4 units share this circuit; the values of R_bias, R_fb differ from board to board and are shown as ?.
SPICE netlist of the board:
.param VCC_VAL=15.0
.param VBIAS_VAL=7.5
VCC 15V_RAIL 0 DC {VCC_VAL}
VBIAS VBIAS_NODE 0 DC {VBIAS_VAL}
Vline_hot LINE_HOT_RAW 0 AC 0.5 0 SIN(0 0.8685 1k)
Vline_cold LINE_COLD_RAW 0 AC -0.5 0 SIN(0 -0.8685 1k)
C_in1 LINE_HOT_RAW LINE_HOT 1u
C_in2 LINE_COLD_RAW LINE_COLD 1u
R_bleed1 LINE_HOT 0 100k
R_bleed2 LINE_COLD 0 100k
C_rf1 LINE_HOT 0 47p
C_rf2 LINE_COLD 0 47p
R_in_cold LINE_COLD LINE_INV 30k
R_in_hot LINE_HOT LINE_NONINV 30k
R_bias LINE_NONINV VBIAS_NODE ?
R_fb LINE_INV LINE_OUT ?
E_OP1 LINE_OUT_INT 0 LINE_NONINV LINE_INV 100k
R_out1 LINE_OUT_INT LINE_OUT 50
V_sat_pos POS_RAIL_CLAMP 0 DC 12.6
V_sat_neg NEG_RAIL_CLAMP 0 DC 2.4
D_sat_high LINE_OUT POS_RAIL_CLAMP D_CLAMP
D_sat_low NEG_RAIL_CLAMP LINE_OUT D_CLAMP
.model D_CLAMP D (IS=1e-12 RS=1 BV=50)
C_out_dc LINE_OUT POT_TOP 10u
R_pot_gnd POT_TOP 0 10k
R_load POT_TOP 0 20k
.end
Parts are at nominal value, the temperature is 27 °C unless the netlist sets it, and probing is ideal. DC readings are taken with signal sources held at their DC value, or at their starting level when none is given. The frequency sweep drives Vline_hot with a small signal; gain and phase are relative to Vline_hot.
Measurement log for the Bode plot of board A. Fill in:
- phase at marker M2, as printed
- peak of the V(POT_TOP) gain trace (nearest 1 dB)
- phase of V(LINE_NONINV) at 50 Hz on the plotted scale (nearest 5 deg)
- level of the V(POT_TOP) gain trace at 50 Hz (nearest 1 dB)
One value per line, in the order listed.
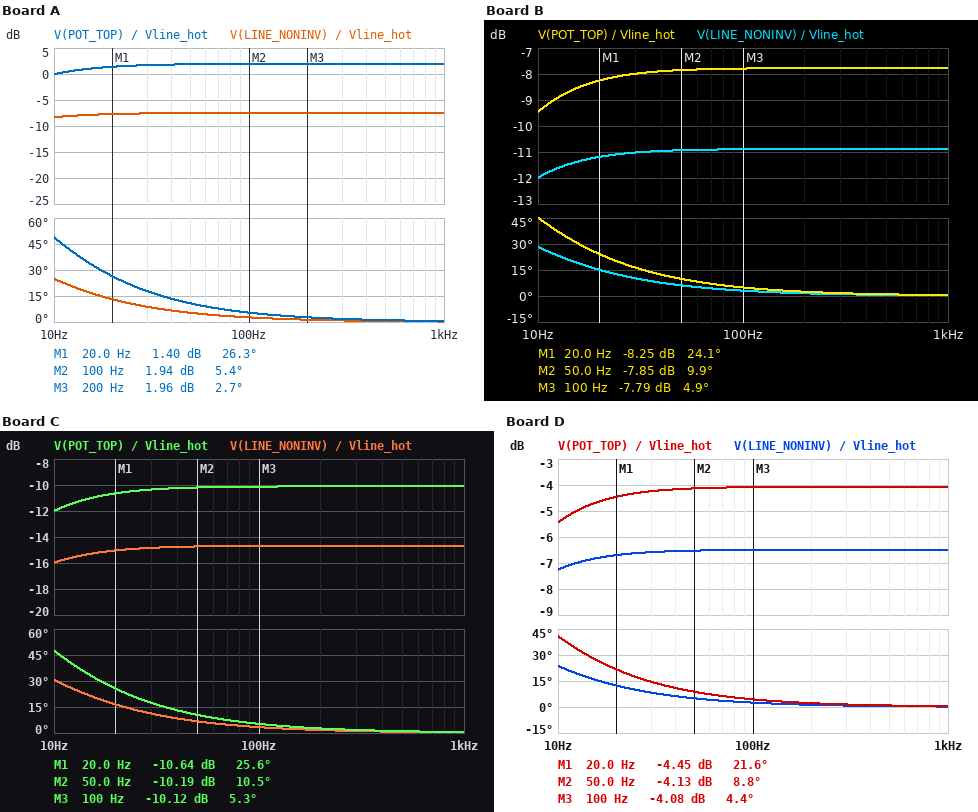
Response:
5.4 deg
2 dB
5 deg
2 dB
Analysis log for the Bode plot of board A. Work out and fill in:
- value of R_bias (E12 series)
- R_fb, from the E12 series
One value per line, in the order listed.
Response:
22 kΩ
27 kΩ
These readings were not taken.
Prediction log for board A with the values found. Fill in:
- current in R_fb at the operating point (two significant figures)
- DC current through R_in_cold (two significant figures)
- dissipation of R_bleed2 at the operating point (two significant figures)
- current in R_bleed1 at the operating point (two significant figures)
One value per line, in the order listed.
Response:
49 µA
49 µA
240 µW
49 µA
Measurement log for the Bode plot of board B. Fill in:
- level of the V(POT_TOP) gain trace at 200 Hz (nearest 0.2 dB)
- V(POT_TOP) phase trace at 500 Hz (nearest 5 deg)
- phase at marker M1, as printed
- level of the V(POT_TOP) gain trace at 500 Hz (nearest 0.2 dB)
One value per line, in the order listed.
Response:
-7.8 dB
0 deg
24.1 deg
-7.8 dB
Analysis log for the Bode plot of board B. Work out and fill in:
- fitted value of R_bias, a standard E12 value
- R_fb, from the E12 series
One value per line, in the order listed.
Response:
12 kΩ
4.7 kΩ
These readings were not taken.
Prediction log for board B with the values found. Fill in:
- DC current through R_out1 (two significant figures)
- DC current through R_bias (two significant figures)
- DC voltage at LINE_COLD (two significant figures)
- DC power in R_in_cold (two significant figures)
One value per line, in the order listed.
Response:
53 µA
53 µA
5.3 V
84 µW
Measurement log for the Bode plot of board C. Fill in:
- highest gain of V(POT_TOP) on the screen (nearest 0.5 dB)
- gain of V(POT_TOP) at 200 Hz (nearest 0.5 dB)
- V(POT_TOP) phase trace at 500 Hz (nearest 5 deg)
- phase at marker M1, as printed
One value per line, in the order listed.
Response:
-10.0 dB
-10.0 dB
0 deg
25.6 deg
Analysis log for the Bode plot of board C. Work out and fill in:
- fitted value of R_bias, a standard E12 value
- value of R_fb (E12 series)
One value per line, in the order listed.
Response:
6.8 kΩ
5.6 kΩ
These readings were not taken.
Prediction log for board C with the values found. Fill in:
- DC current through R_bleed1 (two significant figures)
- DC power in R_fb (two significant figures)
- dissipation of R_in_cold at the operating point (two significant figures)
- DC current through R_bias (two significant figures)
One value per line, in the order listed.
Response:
55 µA
17 µW
90 µW
55 µA
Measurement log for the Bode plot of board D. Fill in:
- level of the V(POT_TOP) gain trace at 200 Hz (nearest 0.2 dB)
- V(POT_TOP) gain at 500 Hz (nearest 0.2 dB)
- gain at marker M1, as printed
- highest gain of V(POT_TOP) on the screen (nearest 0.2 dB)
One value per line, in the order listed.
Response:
-4.0 dB
-4.0 dB
-4.45 dB
-4.0 dB
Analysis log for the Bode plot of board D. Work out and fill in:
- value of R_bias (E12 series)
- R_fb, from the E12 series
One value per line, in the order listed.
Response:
27 kΩ
4.7 kΩ
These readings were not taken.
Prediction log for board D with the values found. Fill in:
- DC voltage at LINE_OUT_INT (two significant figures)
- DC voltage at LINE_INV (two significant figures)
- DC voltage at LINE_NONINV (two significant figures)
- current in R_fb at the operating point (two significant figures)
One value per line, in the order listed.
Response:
6.4 V
6.2 V
6.2 V
48 µA
